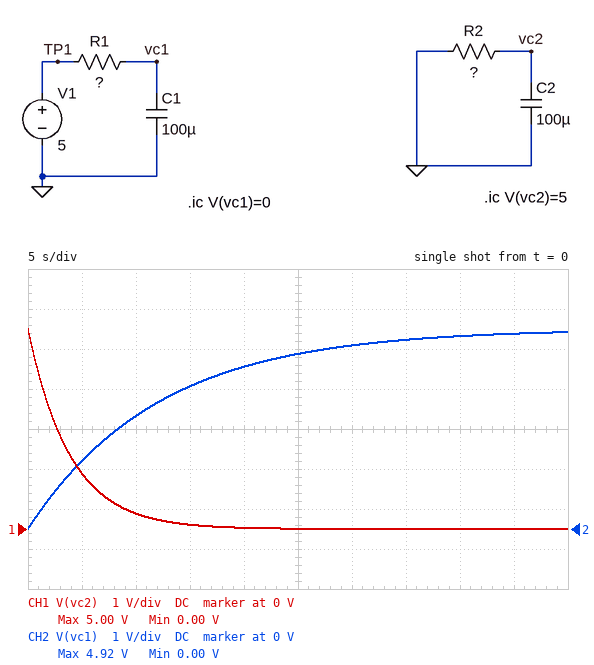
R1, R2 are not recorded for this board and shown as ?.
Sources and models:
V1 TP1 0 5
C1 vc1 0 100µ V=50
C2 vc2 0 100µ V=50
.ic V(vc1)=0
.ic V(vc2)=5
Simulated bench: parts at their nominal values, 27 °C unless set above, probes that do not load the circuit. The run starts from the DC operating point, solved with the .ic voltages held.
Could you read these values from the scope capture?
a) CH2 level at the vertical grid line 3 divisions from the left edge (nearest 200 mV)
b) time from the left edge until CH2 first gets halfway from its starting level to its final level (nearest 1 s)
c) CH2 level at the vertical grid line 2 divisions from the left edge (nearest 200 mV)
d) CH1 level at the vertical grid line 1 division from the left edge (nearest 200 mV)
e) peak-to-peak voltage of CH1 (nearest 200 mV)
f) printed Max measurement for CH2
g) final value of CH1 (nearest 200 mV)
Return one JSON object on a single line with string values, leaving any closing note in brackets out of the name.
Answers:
{"CH2 level at the vertical grid line 3 divisions from the left edge": "3.6 V", "time from the left edge until CH2 first gets halfway from its starting level to its final level": "8 s", "CH2 level at the vertical grid line 2 divisions from the left edge": "2.8 V", "CH1 level at the vertical grid line 1 division from the left edge": "1.4 V", "peak-to-peak voltage of CH1": "5.0 V", "printed Max measurement for CH2": "4.92 V", "final value of CH1": "0 V"}
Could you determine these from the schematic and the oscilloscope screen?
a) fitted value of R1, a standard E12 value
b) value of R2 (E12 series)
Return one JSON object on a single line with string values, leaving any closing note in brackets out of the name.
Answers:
{"fitted value of R1, a standard E12 value": "120 kΩ", "value of R2": "39 kΩ"}
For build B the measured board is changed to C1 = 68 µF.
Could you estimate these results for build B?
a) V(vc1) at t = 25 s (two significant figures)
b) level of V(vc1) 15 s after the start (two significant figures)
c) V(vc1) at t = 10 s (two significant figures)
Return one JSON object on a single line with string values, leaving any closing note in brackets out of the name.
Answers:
{"V(vc1) at t = 25 s": "4.8 V", "level of V(vc1) 15 s after the start": "4.2 V", "V(vc1) at t = 10 s": "3.5 V"}
